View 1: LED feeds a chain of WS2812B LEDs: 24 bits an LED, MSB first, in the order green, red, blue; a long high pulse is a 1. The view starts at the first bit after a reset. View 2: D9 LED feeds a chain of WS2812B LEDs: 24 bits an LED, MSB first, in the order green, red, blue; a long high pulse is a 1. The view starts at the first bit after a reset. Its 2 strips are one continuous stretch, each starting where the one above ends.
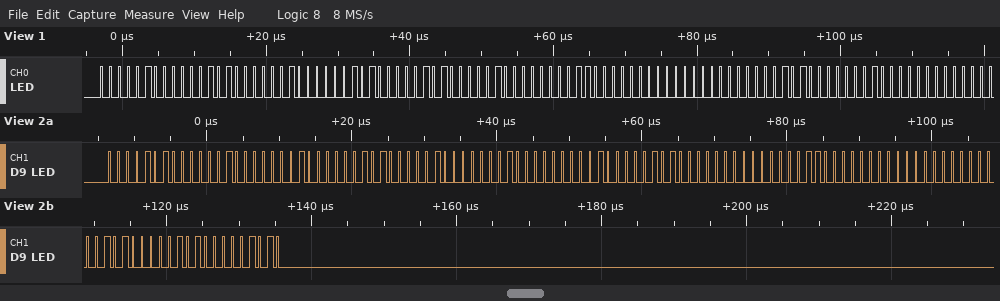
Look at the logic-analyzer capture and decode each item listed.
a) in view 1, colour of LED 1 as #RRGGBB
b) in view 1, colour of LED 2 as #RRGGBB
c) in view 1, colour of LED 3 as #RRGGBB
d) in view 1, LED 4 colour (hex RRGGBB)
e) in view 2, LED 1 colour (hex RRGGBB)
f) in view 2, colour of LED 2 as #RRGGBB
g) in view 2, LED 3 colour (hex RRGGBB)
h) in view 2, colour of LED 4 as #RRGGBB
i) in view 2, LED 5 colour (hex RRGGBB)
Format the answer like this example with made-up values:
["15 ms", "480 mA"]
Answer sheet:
["#0A0404", "#0A0A08", "#000600", "#020A00", "#040A04", "#080A08", "#0A0200", "#000600", "#0A0A0A"]
